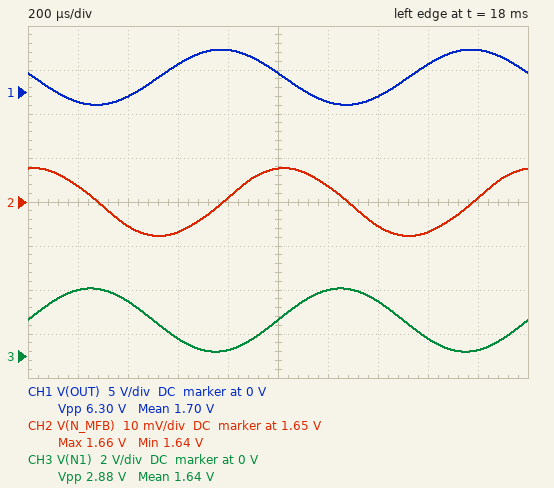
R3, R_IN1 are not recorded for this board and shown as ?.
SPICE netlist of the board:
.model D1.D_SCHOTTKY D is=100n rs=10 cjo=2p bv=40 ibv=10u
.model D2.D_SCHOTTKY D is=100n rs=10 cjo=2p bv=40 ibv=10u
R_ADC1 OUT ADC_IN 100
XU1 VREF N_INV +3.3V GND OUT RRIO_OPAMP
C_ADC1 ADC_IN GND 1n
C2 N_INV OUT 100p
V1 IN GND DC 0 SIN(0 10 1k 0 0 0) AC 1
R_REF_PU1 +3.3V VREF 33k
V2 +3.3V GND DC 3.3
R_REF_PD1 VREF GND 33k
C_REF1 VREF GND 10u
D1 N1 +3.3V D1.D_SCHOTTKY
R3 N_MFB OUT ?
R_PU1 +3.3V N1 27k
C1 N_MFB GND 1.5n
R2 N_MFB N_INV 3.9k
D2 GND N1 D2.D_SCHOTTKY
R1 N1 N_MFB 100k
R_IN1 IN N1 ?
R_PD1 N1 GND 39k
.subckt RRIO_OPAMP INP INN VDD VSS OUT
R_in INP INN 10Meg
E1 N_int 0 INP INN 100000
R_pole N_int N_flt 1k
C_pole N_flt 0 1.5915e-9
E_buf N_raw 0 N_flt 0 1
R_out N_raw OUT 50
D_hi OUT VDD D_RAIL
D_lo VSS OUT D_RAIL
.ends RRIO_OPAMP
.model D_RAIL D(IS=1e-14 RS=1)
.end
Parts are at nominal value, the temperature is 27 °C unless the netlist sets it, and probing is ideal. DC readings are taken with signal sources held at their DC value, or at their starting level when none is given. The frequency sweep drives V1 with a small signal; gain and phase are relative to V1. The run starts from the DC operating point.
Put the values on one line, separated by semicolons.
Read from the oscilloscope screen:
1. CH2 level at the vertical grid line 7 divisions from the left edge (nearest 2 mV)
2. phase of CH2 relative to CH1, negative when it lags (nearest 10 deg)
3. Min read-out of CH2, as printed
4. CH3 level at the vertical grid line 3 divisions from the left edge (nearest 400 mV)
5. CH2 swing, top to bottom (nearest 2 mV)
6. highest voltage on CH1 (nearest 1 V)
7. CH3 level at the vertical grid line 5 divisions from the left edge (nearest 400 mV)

1.644 V; -90 deg; 1.64 V; 800 mV; 16 mV; 5 V; 1.6 V
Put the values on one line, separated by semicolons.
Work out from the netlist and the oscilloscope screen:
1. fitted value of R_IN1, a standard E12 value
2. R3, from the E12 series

82 kΩ; 220 kΩ
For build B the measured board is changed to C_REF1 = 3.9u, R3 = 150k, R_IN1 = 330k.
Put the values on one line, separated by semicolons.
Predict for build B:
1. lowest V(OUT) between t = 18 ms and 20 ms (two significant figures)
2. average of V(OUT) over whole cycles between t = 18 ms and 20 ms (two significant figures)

780 mV; 1.4 V
